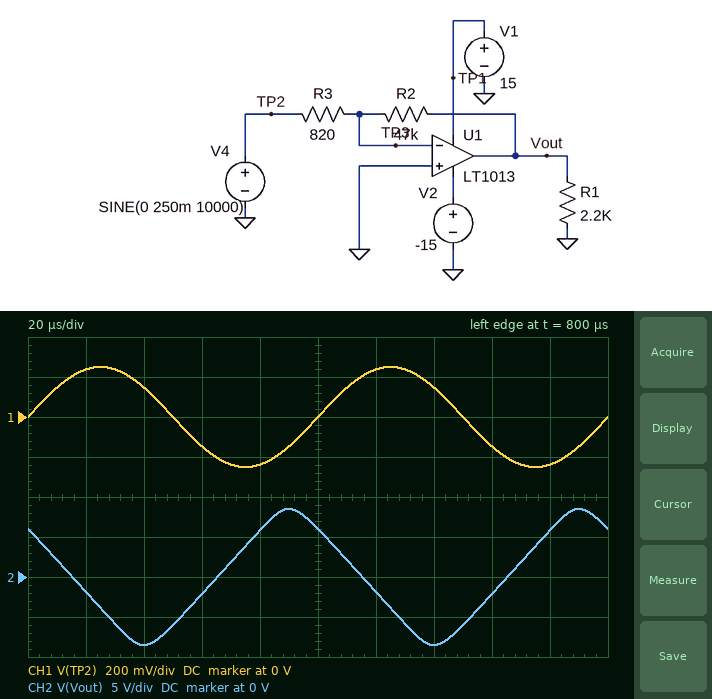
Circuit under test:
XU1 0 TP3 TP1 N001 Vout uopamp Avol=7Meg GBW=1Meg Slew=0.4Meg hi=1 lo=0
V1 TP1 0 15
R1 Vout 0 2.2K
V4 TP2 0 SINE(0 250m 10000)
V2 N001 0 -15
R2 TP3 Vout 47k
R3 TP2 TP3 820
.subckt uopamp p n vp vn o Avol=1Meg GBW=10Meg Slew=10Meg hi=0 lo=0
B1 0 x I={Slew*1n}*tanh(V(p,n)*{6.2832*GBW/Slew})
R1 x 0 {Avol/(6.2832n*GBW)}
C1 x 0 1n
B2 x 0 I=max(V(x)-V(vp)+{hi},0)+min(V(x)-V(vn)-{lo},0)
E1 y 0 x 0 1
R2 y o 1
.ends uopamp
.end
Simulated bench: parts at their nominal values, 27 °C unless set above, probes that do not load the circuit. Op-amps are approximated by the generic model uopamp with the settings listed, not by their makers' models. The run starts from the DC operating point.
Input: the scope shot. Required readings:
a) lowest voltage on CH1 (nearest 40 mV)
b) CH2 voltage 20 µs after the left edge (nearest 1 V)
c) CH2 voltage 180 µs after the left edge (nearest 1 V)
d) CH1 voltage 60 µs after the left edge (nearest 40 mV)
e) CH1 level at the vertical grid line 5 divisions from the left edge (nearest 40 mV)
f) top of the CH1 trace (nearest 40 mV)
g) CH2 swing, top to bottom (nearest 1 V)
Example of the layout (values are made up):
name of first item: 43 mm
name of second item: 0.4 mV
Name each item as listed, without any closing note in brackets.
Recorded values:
lowest voltage on CH1: -240 mV
CH2 voltage 20 µs after the left edge: -2 V
CH2 voltage 180 µs after the left edge: 6 V
CH1 voltage 60 µs after the left edge: -160 mV
CH1 level at the vertical grid line 5 divisions from the left edge: 0 V
top of the CH1 trace: 240 mV
CH2 swing, top to bottom: 17 V
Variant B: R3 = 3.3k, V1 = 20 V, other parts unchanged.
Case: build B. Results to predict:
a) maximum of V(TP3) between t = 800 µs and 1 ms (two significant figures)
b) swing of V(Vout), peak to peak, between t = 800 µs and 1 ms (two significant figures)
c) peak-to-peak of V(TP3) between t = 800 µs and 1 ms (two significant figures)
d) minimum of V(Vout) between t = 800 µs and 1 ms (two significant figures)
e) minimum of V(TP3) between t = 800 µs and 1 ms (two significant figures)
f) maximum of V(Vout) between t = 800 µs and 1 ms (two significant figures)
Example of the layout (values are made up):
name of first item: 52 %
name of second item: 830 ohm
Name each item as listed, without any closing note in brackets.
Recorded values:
maximum of V(TP3) between t = 800 µs and 1 ms: 39 mV
swing of V(Vout), peak to peak, between t = 800 µs and 1 ms: 7.0 V
peak-to-peak of V(TP3) between t = 800 µs and 1 ms: 78 mV
minimum of V(Vout) between t = 800 µs and 1 ms: -3.5 V
minimum of V(TP3) between t = 800 µs and 1 ms: -39 mV
maximum of V(Vout) between t = 800 µs and 1 ms: 3.5 V
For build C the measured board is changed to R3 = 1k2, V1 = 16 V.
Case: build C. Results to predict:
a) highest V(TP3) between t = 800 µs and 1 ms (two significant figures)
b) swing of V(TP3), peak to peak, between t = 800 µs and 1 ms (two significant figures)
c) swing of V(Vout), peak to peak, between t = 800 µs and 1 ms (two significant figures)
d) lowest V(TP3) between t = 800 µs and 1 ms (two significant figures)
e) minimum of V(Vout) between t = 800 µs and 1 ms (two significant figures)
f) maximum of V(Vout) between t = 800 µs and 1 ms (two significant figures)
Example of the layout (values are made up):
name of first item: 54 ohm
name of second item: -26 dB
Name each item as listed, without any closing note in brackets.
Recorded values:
highest V(TP3) between t = 800 µs and 1 ms: 160 mV
swing of V(TP3), peak to peak, between t = 800 µs and 1 ms: 310 mV
swing of V(Vout), peak to peak, between t = 800 µs and 1 ms: 16 V
lowest V(TP3) between t = 800 µs and 1 ms: -160 mV
minimum of V(Vout) between t = 800 µs and 1 ms: -7.9 V
maximum of V(Vout) between t = 800 µs and 1 ms: 7.9 V
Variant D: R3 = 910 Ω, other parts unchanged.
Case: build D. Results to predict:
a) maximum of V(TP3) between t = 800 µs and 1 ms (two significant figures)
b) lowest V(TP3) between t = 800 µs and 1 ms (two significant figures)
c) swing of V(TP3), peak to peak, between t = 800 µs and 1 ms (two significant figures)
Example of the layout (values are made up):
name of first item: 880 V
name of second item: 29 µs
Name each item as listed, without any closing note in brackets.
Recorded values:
maximum of V(TP3) between t = 800 µs and 1 ms: 190 mV
lowest V(TP3) between t = 800 µs and 1 ms: -190 mV
swing of V(TP3), peak to peak, between t = 800 µs and 1 ms: 390 mV
